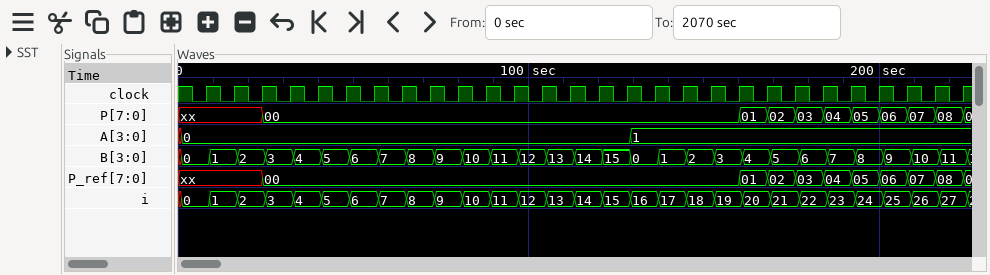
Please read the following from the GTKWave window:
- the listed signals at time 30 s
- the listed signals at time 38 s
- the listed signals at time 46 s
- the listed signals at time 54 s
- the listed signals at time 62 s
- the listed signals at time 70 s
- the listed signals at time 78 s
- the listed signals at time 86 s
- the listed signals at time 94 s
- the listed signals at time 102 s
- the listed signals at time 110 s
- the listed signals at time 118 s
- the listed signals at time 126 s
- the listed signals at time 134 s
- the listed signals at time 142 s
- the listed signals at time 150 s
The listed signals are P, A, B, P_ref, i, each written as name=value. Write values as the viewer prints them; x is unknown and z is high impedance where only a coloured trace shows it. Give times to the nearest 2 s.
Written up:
P=00, A=0, B=3, P_ref=00, i=3
P=00, A=0, B=4, P_ref=00, i=4
P=00, A=0, B=5, P_ref=00, i=5
P=00, A=0, B=6, P_ref=00, i=6
P=00, A=0, B=7, P_ref=00, i=7
P=00, A=0, B=8, P_ref=00, i=8
P=00, A=0, B=9, P_ref=00, i=9
P=00, A=0, B=10, P_ref=00, i=10
P=00, A=0, B=11, P_ref=00, i=11
P=00, A=0, B=12, P_ref=00, i=12
P=00, A=0, B=13, P_ref=00, i=13
P=00, A=0, B=14, P_ref=00, i=14
P=00, A=0, B=15, P_ref=00, i=15
P=00, A=1, B=0, P_ref=00, i=16
P=00, A=1, B=1, P_ref=00, i=17
P=00, A=1, B=2, P_ref=00, i=18
